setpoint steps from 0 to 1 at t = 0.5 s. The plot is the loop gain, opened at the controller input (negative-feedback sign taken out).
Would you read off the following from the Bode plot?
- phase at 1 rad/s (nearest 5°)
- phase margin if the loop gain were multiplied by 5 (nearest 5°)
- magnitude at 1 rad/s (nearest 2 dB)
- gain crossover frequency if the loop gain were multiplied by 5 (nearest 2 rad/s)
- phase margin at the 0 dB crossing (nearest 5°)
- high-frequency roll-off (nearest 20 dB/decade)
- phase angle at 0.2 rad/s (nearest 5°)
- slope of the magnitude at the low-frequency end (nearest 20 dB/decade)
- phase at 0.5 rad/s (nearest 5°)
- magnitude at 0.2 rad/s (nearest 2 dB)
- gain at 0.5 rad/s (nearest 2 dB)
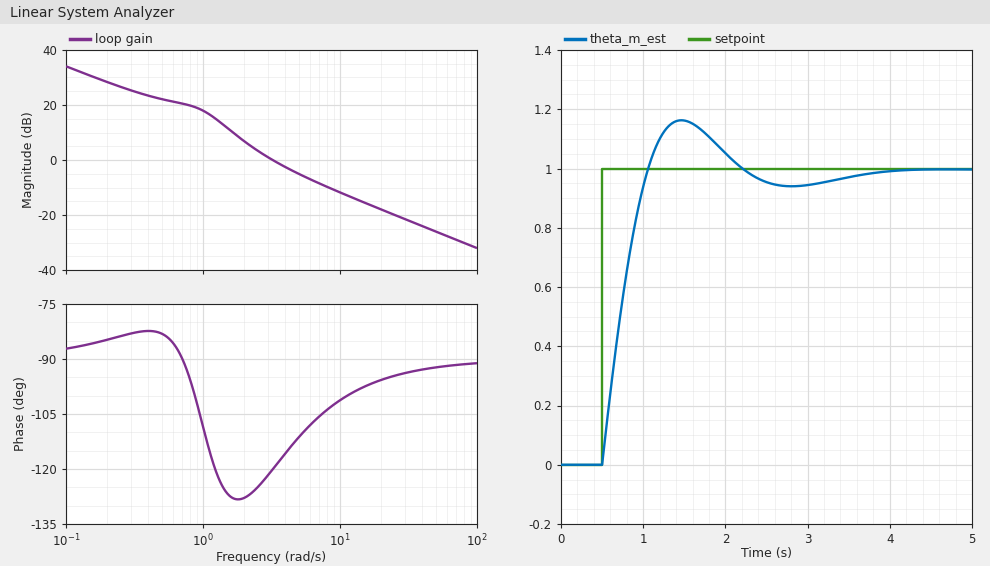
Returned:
-110°
80°
18 dB
12 rad/s
60°
-20 dB/decade
-85°
-20 dB/decade
-85°
28 dB
22 dB
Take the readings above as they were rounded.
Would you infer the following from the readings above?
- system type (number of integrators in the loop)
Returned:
1
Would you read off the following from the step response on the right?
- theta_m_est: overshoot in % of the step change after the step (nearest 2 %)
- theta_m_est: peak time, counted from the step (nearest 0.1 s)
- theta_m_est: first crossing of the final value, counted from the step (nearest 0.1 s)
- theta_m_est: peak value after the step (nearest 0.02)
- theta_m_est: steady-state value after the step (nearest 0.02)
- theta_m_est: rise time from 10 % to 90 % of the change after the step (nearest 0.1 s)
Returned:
16 %
1.0 s
0.6 s
1.16
1.00
0.4 s
